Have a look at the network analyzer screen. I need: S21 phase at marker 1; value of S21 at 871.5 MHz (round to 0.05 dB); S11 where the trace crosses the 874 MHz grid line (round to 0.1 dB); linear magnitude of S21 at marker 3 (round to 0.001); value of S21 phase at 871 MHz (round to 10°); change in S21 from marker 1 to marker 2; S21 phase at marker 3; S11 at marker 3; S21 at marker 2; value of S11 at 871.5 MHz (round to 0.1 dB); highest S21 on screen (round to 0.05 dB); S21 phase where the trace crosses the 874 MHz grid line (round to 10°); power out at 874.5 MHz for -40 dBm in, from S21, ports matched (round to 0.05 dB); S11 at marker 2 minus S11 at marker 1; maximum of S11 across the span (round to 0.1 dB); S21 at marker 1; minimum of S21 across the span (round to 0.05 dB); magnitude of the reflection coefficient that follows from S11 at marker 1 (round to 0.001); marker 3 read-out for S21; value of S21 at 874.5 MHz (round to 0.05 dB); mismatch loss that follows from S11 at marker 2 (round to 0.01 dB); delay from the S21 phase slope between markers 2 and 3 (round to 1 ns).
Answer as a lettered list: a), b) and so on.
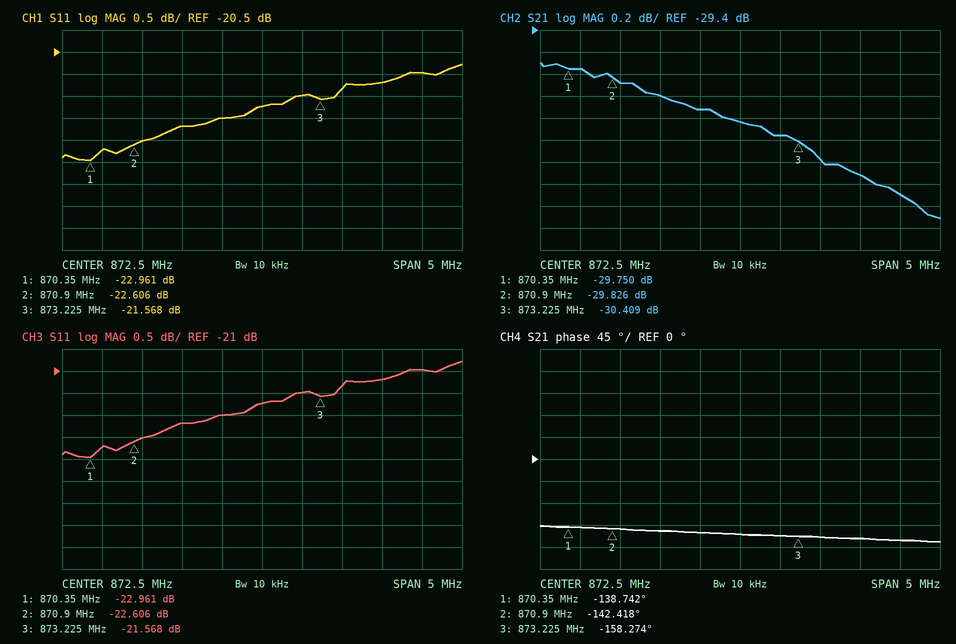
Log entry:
a) -138.742°
b) -30.00 dB
c) -21.2 dB
d) 0.030
e) -140°
f) -0.076 dB
g) -158.274°
h) -21.568 dB
i) -29.826 dB
j) -22.2 dB
k) -29.70 dB
l) -160°
m) -70.90 dBm
n) 0.355 dB
o) -20.8 dB
p) -29.750 dB
q) -31.10 dB
r) 0.071
s) -30.409 dB
t) -30.90 dB
u) 0.02 dB
v) 19 ns
